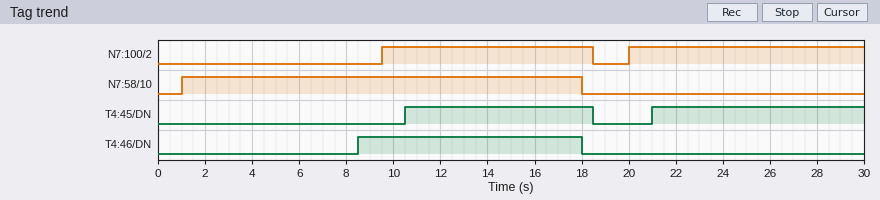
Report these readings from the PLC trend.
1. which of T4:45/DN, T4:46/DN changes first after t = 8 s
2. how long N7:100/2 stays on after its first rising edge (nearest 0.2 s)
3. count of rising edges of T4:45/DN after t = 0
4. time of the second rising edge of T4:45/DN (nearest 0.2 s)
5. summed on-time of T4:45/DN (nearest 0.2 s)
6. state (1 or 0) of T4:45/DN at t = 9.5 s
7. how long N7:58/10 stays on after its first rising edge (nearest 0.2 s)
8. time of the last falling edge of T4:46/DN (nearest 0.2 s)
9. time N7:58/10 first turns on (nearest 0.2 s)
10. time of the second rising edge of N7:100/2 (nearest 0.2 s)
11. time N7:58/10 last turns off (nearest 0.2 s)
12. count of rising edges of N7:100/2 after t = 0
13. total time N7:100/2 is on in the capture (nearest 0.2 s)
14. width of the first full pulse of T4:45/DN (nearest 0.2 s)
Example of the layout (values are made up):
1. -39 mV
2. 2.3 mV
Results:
1. T4:46/DN
2. 9.0 s
3. 2
4. 21.0 s
5. 17.0 s
6. 0
7. 17.0 s
8. 18.0 s
9. 1.0 s
10. 20.0 s
11. 18.0 s
12. 2
13. 19.0 s
14. 8.0 s
